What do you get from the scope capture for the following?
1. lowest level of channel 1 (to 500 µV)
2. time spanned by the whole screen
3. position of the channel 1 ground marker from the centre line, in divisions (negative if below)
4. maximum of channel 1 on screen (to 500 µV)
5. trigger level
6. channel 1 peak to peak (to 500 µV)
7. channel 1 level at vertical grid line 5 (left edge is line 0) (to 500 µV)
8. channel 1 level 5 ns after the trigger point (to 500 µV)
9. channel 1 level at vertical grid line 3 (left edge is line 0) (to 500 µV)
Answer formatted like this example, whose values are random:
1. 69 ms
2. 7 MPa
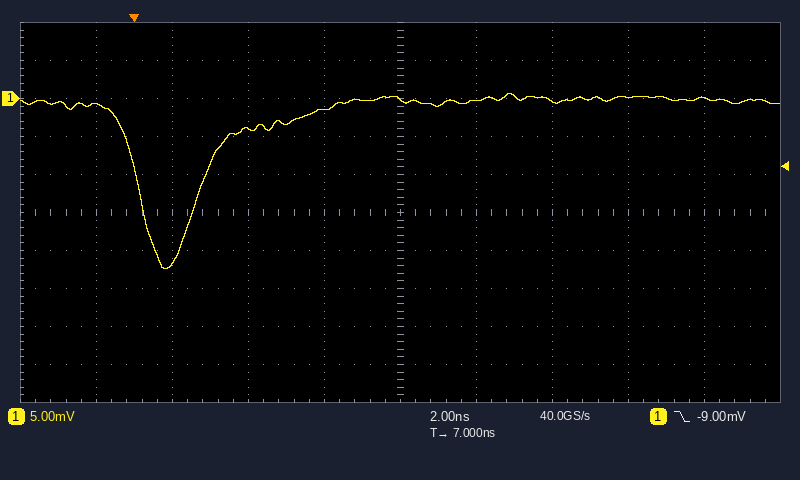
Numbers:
1. -22.5 mV
2. 20 ns
3. +3.0 div
4. 500 µV
5. -9.00 mV
6. 23.0 mV
7. 0.0 mV
8. -1.5 mV
9. -4.0 mV
